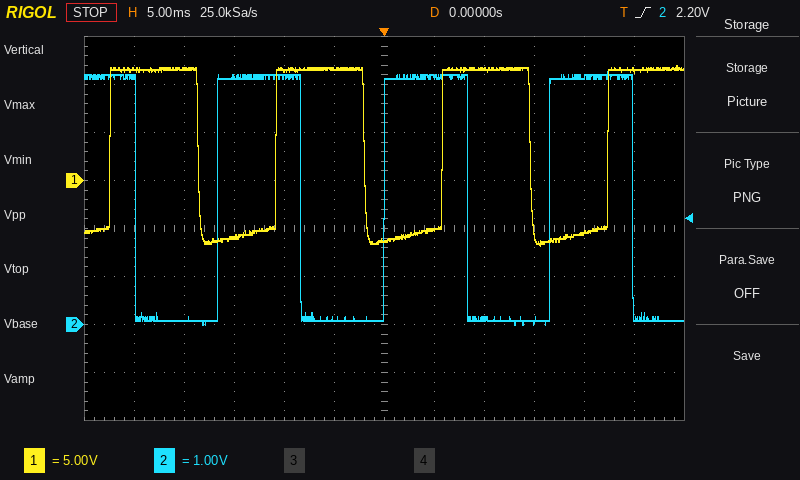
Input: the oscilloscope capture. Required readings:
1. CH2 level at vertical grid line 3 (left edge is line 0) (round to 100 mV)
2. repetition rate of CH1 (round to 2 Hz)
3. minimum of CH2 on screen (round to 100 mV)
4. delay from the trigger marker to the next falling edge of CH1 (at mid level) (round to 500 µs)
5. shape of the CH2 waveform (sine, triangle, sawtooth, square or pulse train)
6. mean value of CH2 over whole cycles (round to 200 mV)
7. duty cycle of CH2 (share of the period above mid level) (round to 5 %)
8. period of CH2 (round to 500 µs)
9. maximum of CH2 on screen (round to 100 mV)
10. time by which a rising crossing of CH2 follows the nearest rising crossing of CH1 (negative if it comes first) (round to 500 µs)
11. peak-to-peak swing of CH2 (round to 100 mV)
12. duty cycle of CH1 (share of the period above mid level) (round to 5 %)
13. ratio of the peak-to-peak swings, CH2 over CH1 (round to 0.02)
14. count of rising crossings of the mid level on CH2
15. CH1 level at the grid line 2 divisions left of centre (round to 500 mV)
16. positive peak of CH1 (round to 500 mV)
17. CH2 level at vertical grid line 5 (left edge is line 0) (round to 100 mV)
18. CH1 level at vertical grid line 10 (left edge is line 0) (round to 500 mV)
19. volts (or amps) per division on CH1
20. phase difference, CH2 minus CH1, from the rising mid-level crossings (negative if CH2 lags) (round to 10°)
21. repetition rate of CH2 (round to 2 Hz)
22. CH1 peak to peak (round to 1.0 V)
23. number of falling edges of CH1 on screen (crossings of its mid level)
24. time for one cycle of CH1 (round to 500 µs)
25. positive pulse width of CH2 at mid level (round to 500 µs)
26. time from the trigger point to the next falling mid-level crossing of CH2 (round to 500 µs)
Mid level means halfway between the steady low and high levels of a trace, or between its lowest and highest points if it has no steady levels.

5.2 V
60 Hz
0.0 V
14.5 ms
square
2.6 V
50 %
16.5 ms
5.3 V
-6.0 ms
5.3 V
55 %
0.28
3
11.5 V
12.0 V
100 mV
-5.5 V
5 V
+130°
60 Hz
19.0 V
3
16.5 ms
8.5 ms
8.5 ms
